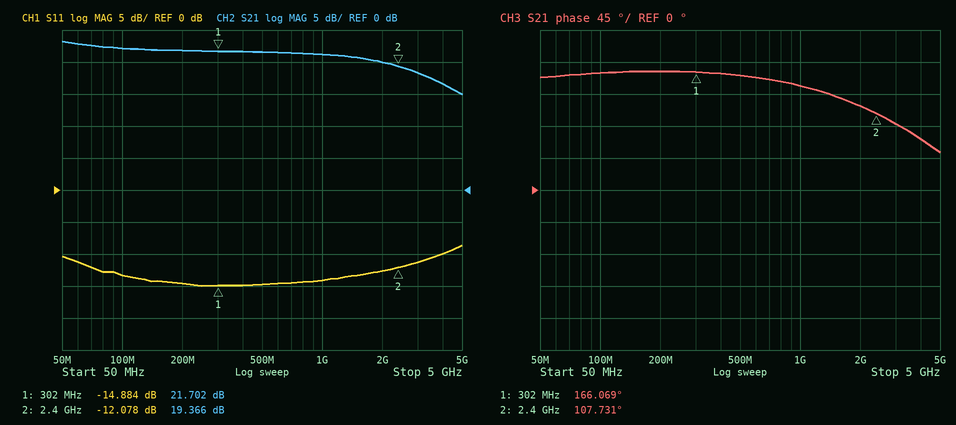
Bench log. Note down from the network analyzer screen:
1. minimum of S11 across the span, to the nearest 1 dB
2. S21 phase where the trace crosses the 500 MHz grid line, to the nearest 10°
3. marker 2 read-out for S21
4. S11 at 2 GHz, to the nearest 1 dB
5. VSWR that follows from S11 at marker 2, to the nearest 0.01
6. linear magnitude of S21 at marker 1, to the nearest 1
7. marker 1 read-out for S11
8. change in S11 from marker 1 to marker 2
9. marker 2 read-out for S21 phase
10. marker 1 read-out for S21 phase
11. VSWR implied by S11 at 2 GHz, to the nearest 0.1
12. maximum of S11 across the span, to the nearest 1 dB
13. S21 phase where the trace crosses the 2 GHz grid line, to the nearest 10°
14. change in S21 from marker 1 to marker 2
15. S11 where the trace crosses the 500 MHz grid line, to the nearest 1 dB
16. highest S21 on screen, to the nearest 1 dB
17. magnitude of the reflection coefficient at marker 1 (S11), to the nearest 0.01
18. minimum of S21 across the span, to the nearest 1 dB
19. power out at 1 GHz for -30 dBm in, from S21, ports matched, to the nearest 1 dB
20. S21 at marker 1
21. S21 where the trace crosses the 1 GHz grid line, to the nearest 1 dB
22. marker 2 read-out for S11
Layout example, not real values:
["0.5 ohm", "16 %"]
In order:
["-15 dB", "160°", "19.366 dB", "-13 dB", "1.66", "12", "-14.884 dB", "2.806 dB", "107.731°", "166.069°", "1.6", "-9 dB", "120°", "-2.336 dB", "-15 dB", "23 dB", "0.18", "15 dB", "-9 dBm", "21.702 dB", "21 dB", "-12.078 dB"]
